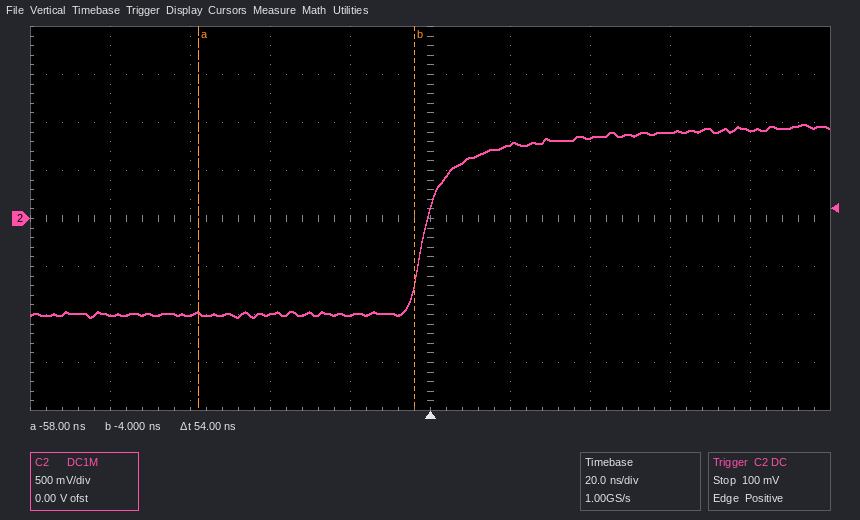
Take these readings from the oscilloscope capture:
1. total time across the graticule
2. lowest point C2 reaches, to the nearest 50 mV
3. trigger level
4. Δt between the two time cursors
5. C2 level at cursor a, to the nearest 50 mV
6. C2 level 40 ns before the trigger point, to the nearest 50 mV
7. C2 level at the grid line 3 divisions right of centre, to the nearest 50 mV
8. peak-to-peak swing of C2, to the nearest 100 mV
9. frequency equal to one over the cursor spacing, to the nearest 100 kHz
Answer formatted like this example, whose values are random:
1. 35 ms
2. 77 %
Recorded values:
1. 200 ns
2. -1.05 V
3. 100 mV
4. 54 ns
5. -1.00 V
6. -1.00 V
7. 900 mV
8. 2.00 V
9. 18.5 MHz
